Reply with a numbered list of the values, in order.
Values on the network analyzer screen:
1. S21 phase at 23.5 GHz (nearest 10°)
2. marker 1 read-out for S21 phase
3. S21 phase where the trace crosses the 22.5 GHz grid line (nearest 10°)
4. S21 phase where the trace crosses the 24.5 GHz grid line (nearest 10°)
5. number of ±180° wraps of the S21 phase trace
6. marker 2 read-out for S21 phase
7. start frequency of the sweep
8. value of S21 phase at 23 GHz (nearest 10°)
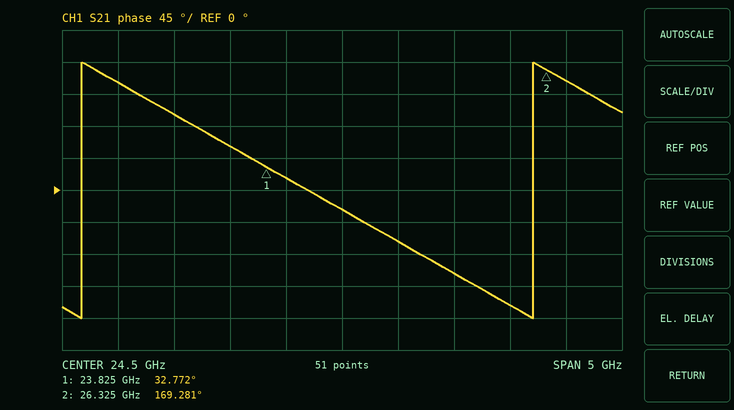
1. 60°
2. 32.772°
3. 150°
4. -30°
5. 2
6. 169.281°
7. 22 GHz
8. 110°
